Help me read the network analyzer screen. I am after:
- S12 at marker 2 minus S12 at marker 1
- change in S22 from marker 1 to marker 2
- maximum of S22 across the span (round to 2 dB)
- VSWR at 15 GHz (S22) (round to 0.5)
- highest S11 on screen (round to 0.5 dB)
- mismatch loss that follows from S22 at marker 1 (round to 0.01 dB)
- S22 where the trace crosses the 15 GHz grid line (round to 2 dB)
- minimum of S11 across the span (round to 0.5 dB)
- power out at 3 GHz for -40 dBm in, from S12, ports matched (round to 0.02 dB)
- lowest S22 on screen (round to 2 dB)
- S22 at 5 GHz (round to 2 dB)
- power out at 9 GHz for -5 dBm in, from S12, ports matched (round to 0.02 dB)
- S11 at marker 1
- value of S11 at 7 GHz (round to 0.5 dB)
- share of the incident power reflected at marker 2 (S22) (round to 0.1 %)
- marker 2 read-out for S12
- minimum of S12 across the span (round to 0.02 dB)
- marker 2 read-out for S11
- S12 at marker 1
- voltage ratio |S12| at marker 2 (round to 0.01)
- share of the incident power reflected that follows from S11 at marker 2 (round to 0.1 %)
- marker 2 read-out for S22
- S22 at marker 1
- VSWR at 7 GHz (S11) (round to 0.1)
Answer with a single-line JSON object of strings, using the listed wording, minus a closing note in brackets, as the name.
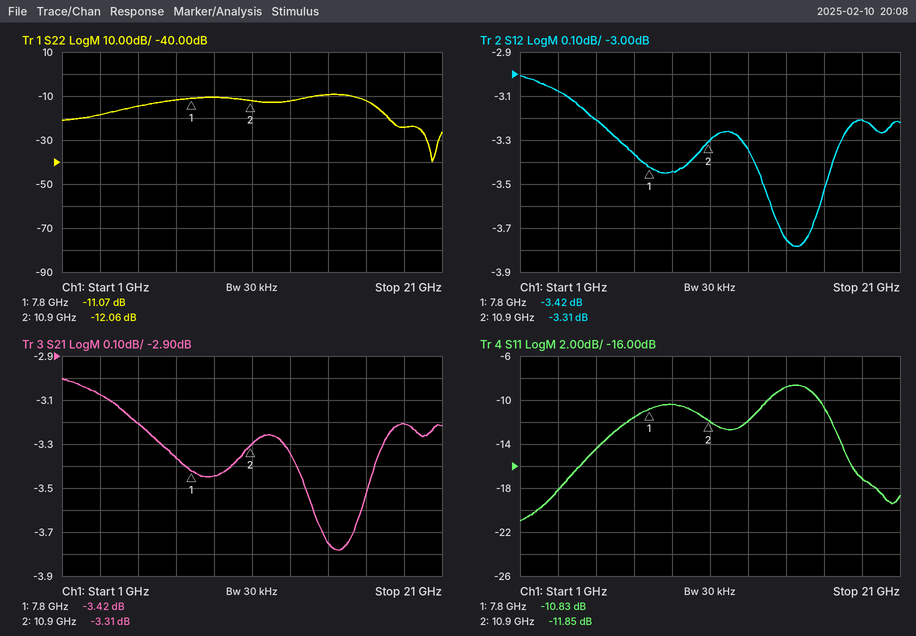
{"S12 at marker 2 minus S12 at marker 1": "0.11 dB", "change in S22 from marker 1 to marker 2": "-0.99 dB", "maximum of S22 across the span": "-10 dB", "VSWR at 15 GHz (S22)": "2.0", "highest S11 on screen": "-8.5 dB", "mismatch loss that follows from S22 at marker 1": "0.35 dB", "S22 where the trace crosses the 15 GHz grid line": "-10 dB", "minimum of S11 across the span": "-21.0 dB", "power out at 3 GHz for -40 dBm in, from S12, ports matched": "-43.08 dBm", "lowest S22 on screen": "-40 dB", "S22 at 5 GHz": "-14 dB", "power out at 9 GHz for -5 dBm in, from S12, ports matched": "-8.44 dBm", "S11 at marker 1": "-10.83 dB", "value of S11 at 7 GHz": "-11.5 dB", "share of the incident power reflected at marker 2 (S22)": "6.2 %", "marker 2 read-out for S12": "-3.31 dB", "minimum of S12 across the span": "-3.78 dB", "marker 2 read-out for S11": "-11.85 dB", "S12 at marker 1": "-3.42 dB", "voltage ratio |S12| at marker 2": "0.68", "share of the incident power reflected that follows from S11 at marker 2": "6.5 %", "marker 2 read-out for S22": "-12.06 dB", "S22 at marker 1": "-11.07 dB", "VSWR at 7 GHz (S11)": "1.7"}
